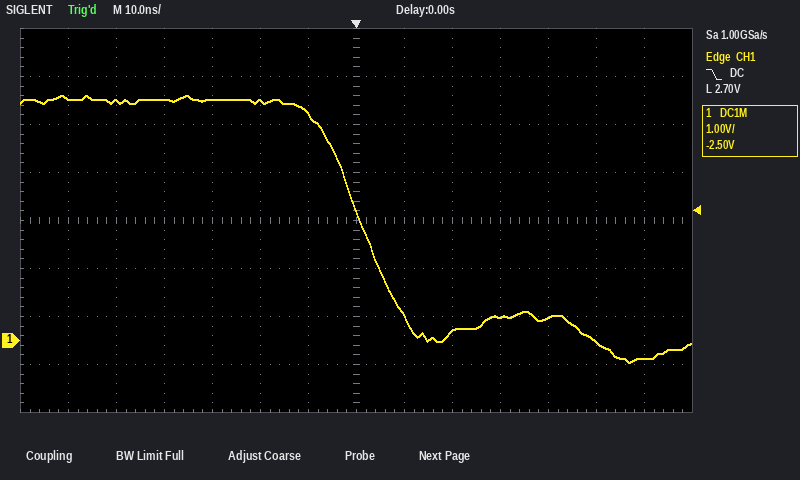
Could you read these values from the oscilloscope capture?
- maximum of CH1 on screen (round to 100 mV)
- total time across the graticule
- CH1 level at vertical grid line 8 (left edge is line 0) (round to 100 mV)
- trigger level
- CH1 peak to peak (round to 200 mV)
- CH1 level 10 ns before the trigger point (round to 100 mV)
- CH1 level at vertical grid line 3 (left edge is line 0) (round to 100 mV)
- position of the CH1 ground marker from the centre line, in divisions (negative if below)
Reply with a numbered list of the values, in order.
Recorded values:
1. 5.1 V
2. 140 ns
3. 500 mV
4. 2.70 V
5. 5.6 V
6. 4.7 V
7. 5.0 V
8. -2.5 div
